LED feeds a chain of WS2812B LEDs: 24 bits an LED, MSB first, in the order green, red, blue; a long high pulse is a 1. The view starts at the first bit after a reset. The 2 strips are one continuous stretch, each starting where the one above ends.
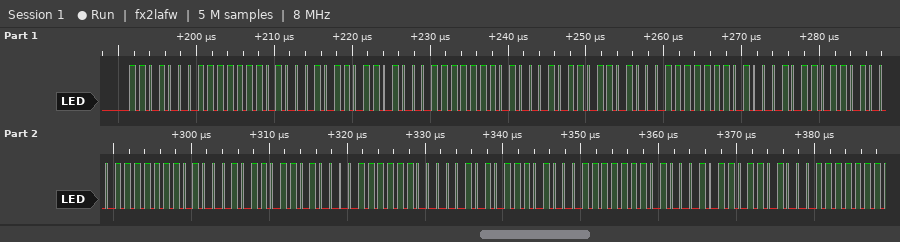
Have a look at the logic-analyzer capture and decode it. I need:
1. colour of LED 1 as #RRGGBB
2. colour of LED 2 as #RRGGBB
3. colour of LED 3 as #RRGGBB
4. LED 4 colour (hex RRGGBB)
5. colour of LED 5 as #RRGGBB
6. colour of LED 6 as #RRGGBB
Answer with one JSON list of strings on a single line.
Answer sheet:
["#FDD116", "#FDD116", "#FDD116", "#FDD116", "#FCD015", "#FDD116"]
